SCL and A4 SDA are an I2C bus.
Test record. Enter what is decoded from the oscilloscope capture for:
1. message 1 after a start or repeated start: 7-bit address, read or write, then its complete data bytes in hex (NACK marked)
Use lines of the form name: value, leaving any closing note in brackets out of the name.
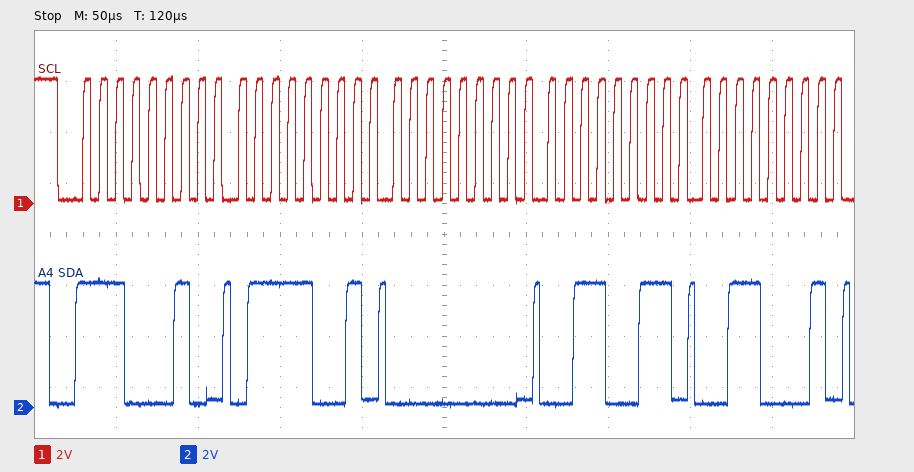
message 1 after a start or repeated start: 7-bit address, read or write, then its complete data bytes in hex: 0x71 write: 79 00 33 31
